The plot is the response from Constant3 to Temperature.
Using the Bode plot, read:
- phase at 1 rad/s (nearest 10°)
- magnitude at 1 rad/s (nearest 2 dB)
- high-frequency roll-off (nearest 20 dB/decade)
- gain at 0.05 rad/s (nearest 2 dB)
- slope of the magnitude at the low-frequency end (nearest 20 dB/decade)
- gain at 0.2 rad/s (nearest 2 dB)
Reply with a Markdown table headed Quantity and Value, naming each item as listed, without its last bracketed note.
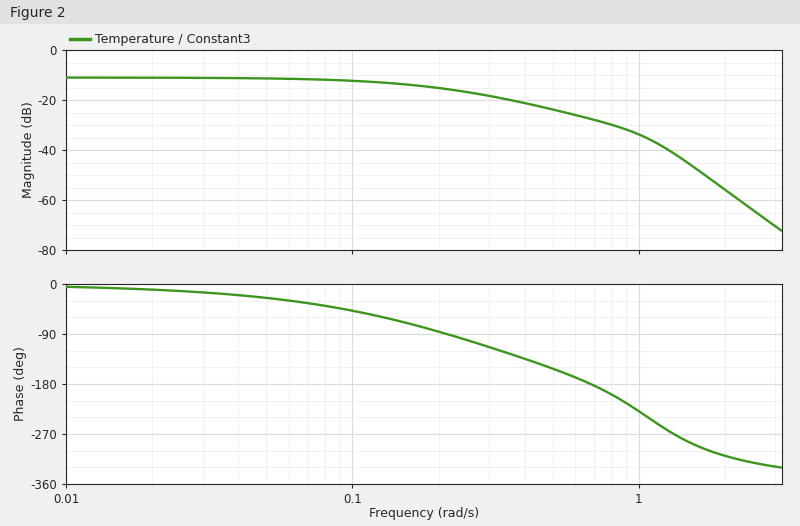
| Quantity | Value |
|---|---|
| phase at 1 rad/s | -230° |
| magnitude at 1 rad/s | -34 dB |
| high-frequency roll-off | -80 dB/decade |
| gain at 0.05 rad/s | -12 dB |
| slope of the magnitude at the low-frequency end | 0 dB/decade |
| gain at 0.2 rad/s | -16 dB |
